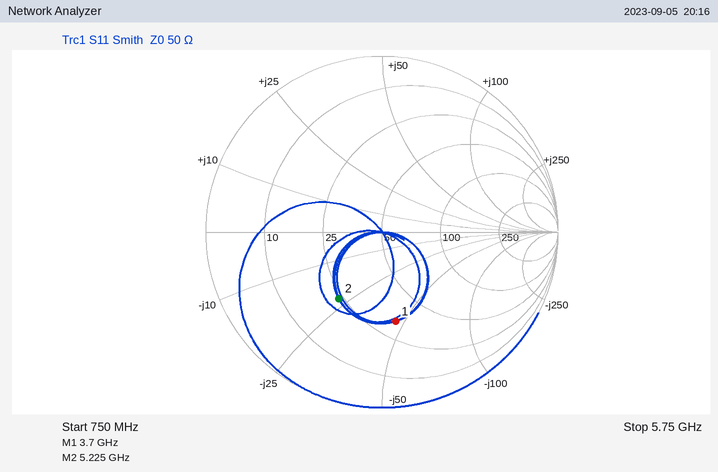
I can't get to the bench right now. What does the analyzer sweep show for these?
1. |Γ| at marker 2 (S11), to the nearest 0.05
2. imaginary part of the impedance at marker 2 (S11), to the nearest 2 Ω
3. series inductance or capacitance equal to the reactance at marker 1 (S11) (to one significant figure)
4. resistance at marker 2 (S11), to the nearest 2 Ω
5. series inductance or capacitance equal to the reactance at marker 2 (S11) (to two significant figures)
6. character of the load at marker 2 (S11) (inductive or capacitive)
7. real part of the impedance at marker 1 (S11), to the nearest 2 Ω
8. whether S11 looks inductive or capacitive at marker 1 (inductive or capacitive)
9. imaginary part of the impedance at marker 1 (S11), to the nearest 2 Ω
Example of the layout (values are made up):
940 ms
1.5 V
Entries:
0.45
-22 Ω
900 fF
24 Ω
1.4 pF
capacitive
34 Ω
capacitive
-46 Ω
